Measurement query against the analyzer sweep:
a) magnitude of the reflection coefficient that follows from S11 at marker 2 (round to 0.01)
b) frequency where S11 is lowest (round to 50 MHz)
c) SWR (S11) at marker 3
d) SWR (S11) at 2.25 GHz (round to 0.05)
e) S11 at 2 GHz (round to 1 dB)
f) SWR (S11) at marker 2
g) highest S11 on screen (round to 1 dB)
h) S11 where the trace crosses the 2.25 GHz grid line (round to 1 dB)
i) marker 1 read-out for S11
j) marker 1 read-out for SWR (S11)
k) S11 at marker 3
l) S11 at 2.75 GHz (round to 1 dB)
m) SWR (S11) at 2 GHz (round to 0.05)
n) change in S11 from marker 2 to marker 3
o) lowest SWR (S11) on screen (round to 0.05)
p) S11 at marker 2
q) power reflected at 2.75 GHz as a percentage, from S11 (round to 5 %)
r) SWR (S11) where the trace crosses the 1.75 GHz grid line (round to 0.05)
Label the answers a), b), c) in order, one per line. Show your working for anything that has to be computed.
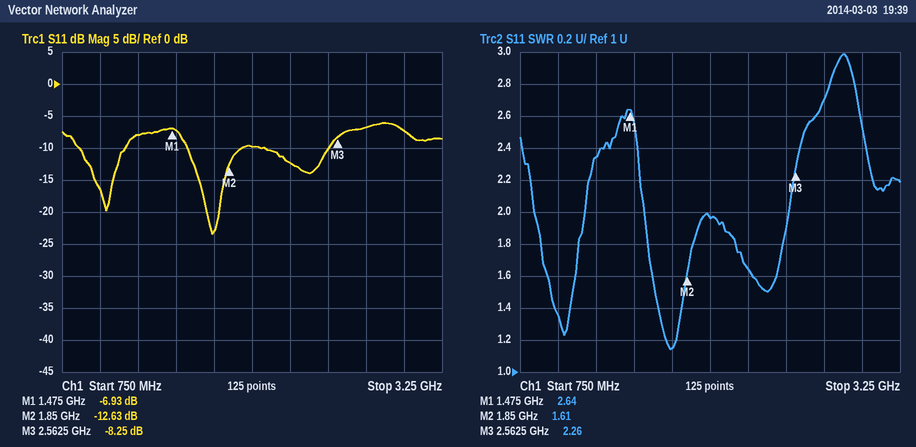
a) 10^(-12.63/20) ≈ 0.23
b) 1.75 GHz
c) 2.26
d) 1.65
e) -10 dB
f) 1.61
g) -6 dB
h) -12 dB
i) -6.93 dB
j) 2.64
k) -8.25 dB
l) -7 dB
m) 1.95
n) -8.25 − (-12.63) = 4.38 dB
o) 1.15
p) -12.63 dB
q) 10^(-7/10) ≈ 20 %
r) 1.15
